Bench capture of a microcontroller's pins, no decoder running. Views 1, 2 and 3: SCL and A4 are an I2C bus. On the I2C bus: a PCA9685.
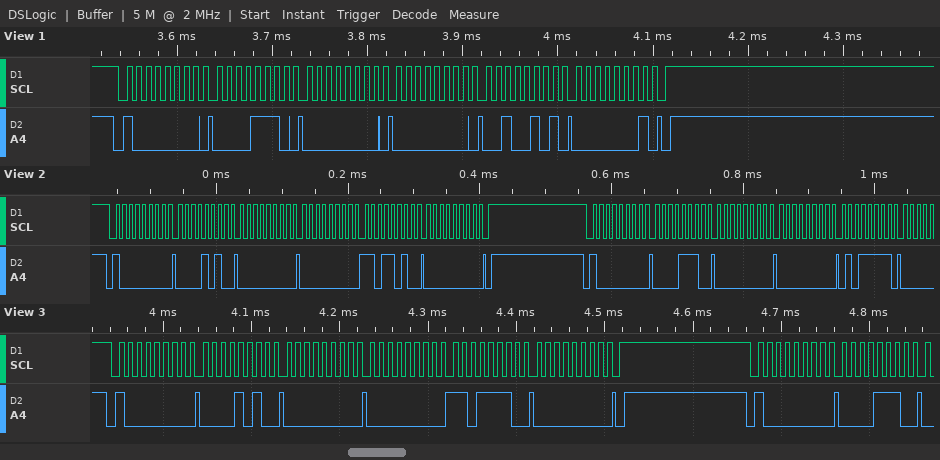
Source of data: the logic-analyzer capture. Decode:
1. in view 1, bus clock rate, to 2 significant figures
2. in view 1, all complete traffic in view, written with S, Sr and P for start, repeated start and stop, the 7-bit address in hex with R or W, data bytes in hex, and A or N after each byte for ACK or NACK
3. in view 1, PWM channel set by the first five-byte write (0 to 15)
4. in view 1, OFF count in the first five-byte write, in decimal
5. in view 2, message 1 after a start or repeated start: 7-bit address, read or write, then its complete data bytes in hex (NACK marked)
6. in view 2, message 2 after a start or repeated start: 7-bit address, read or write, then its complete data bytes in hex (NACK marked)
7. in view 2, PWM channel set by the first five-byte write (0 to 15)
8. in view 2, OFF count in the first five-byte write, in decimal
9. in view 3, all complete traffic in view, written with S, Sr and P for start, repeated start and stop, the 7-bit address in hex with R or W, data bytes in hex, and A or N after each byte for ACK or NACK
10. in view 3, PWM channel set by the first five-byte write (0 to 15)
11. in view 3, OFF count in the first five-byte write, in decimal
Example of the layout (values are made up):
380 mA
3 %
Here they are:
100 kHz
S 40W A 0E A 00 A 00 A 25 A 01 A P
2
293
0x40 write: 0A 00 00 DA 00
0x40 write: 0E 00 00 5F
1
218
S 40W A 0A A 00 A 00 A DE A 00 A P S 40W A 0E A
1
222
